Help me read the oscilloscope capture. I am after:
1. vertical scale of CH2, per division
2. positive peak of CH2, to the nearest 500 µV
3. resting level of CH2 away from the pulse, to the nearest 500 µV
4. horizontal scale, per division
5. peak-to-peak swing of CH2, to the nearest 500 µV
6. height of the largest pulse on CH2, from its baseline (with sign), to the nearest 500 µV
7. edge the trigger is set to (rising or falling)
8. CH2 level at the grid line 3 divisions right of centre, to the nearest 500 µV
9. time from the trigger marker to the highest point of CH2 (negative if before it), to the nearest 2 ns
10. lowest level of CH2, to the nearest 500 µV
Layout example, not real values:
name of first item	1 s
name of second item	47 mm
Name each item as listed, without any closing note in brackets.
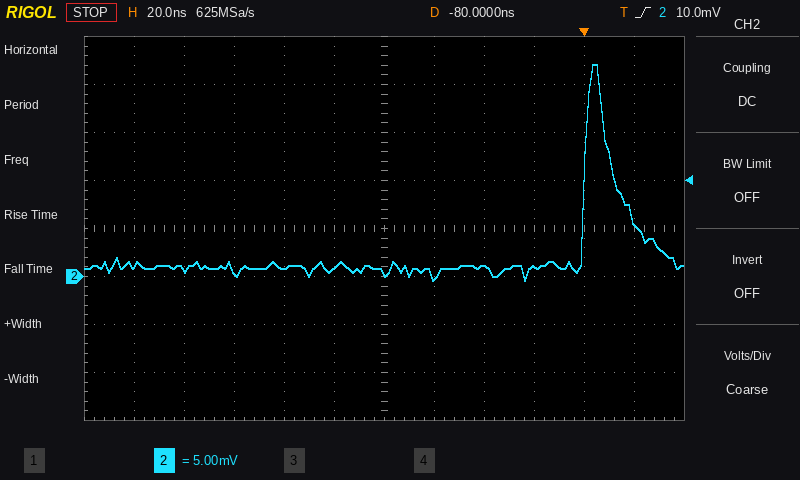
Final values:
vertical scale of CH2, per division	5 mV
positive peak of CH2, to the nearest 500 µV	22.0 mV
resting level of CH2 away from the pulse, to the nearest 500 µV	1.0 mV
horizontal scale, per division	20 ns
peak-to-peak swing of CH2, to the nearest 500 µV	22.5 mV
height of the largest pulse on CH2, from its baseline (with sign), to the nearest 500 µV	+21.0 mV
edge the trigger is set to	rising
CH2 level at the grid line 3 divisions right of centre, to the nearest 500 µV	1.0 mV
time from the trigger marker to the highest point of CH2 (negative if before it), to the nearest 2 ns	+4 ns
lowest level of CH2, to the nearest 500 µV	-500 µV
